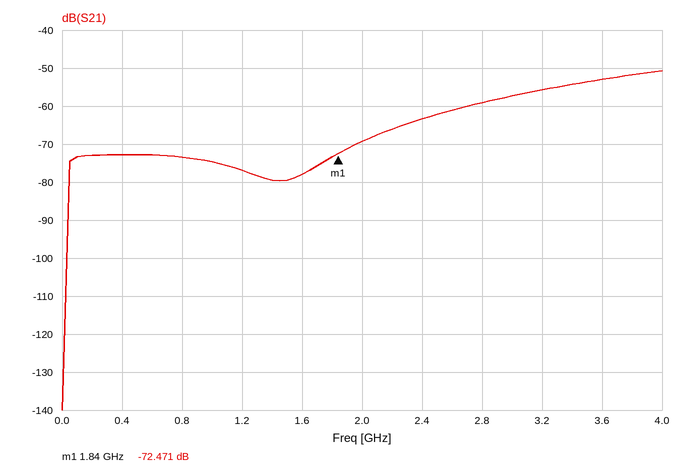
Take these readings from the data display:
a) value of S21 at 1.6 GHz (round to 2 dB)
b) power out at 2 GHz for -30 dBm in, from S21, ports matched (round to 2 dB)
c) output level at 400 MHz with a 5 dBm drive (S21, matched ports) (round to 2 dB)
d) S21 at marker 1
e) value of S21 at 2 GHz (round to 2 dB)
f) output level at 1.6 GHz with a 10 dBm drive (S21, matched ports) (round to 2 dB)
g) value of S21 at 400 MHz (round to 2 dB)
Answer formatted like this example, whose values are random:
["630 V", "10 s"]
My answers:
["-78 dB", "-100 dBm", "-68 dBm", "-72.471 dB", "-70 dB", "-68 dBm", "-72 dB"]
